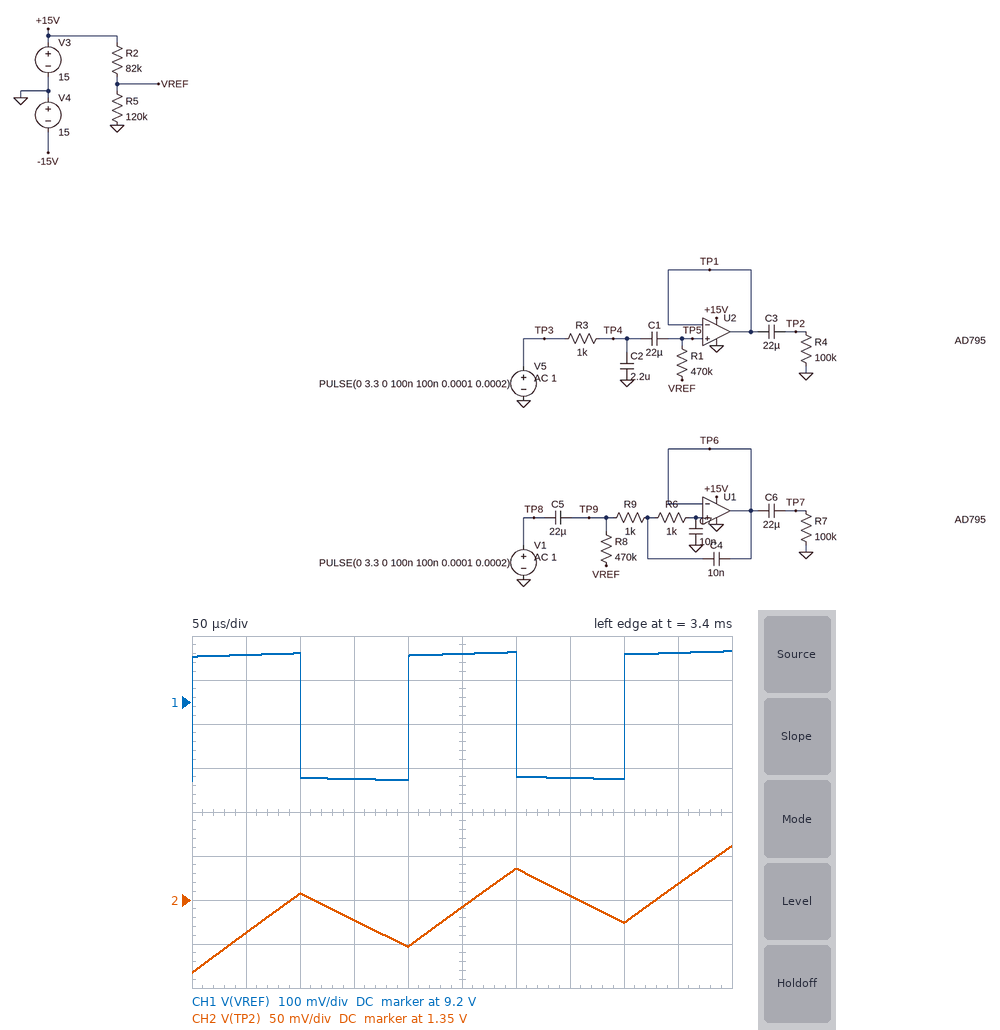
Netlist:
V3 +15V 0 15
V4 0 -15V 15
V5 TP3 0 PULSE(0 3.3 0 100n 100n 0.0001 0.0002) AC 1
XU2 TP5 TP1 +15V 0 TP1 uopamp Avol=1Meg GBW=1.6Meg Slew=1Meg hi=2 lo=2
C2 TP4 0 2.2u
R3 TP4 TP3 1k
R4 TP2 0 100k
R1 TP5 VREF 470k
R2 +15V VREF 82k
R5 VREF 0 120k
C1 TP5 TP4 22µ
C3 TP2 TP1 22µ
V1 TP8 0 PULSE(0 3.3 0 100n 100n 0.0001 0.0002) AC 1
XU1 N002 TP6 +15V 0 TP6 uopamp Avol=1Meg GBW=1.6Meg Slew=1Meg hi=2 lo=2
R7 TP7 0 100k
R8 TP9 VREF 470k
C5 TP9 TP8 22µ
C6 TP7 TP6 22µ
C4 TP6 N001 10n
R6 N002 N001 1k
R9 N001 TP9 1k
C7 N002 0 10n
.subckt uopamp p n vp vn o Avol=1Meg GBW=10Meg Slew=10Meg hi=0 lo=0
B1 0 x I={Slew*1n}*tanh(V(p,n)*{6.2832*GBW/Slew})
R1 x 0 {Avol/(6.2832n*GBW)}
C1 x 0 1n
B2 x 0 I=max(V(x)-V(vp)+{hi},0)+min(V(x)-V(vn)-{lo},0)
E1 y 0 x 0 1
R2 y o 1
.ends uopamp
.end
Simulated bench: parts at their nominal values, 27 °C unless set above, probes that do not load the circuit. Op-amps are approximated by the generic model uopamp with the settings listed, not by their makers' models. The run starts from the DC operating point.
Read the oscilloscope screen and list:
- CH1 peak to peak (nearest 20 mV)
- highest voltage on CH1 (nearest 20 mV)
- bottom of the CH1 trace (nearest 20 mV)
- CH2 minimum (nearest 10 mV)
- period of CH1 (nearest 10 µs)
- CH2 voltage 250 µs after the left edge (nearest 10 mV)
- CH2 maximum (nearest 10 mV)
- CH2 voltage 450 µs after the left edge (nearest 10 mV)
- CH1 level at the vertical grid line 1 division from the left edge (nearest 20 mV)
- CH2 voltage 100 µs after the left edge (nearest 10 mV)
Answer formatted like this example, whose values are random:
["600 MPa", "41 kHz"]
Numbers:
["300 mV", "9.32 V", "9.02 V", "1.27 V", "200 µs", "1.34 V", "1.41 V", "1.37 V", "9.30 V", "1.36 V"]
